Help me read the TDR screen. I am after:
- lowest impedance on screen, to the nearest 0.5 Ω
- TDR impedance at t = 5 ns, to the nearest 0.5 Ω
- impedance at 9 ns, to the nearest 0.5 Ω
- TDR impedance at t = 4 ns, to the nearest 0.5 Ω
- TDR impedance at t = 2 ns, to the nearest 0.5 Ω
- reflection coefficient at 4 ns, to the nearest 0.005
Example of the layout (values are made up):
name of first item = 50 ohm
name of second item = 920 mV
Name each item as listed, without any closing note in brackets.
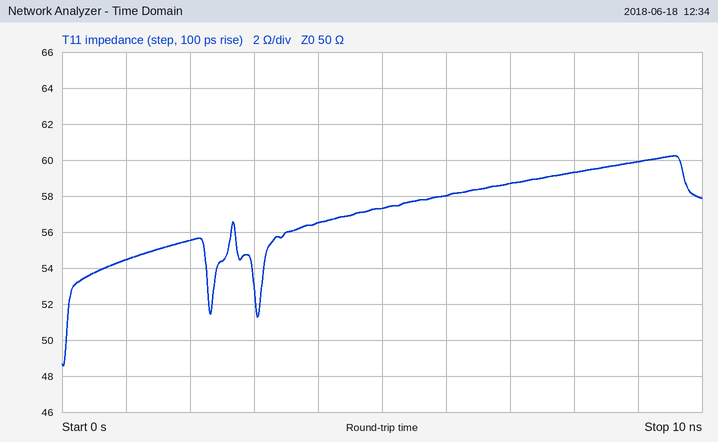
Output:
lowest impedance on screen, to the nearest 0.5 Ω = 48.5 Ω
TDR impedance at t = 5 ns, to the nearest 0.5 Ω = 57.5 Ω
impedance at 9 ns, to the nearest 0.5 Ω = 60.0 Ω
TDR impedance at t = 4 ns, to the nearest 0.5 Ω = 56.5 Ω
TDR impedance at t = 2 ns, to the nearest 0.5 Ω = 55.5 Ω
reflection coefficient at 4 ns, to the nearest 0.005 = +0.060
